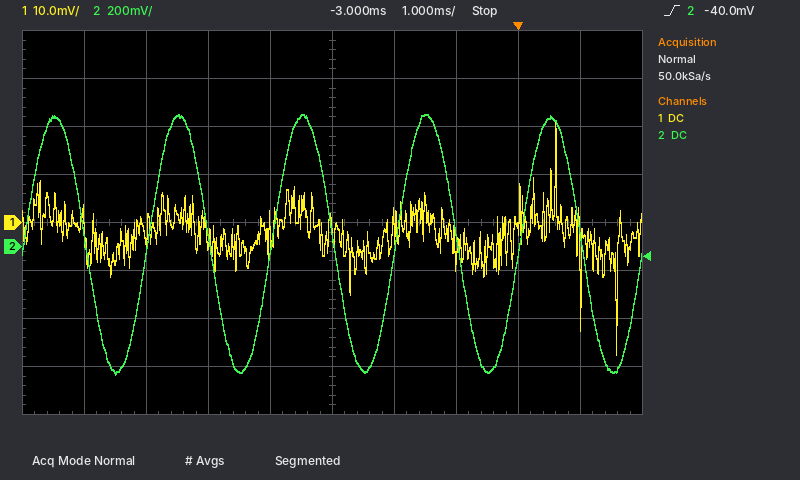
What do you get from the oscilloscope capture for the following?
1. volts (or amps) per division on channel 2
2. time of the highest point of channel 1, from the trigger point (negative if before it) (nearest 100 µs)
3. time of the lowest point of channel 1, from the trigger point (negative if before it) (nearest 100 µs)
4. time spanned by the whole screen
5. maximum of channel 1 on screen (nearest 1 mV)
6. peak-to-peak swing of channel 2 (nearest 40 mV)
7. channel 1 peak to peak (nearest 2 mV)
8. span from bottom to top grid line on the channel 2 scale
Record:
200 mV
+600 µs
+1.6 ms
10 ms
21 mV
1.08 V
48 mV
1.6 V
